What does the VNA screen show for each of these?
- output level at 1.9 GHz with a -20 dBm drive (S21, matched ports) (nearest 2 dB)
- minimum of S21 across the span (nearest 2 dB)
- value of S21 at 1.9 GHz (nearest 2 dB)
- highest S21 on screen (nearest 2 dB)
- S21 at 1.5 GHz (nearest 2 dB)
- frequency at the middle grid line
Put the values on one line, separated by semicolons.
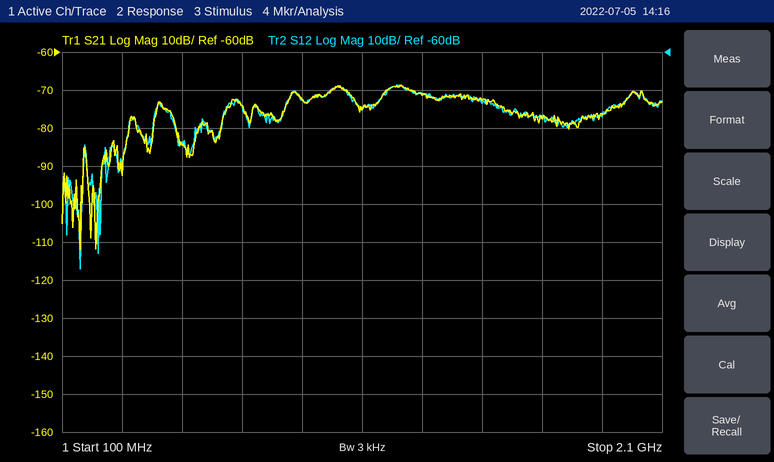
-96 dBm; -112 dB; -76 dB; -68 dB; -72 dB; 1.1 GHz
